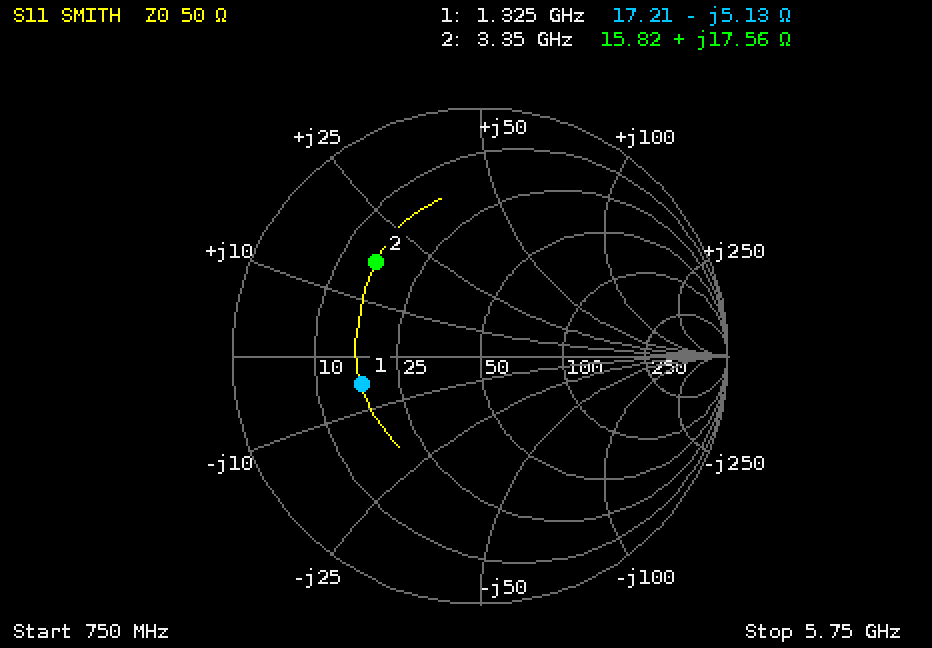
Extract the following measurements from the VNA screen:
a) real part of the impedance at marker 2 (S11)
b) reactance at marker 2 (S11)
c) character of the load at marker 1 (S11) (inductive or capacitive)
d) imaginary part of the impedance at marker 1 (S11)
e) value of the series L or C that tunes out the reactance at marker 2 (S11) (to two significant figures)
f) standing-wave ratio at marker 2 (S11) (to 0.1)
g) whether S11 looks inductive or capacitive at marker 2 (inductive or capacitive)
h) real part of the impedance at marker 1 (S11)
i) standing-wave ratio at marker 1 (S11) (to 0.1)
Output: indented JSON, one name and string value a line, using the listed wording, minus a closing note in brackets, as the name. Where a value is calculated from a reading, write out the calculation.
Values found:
{
  "real part of the impedance at marker 2": "15.82 Ω",
  "reactance at marker 2": "+17.56 Ω",
  "character of the load at marker 1 (S11)": "capacitive",
  "imaginary part of the impedance at marker 1": "-5.13 Ω",
  "value of the series L or C that tunes out the reactance at marker 2 (S11)": "C = 1/(2π × 3.35 GHz × 17.56 Ω) ≈ 2.7 pF",
  "standing-wave ratio at marker 2 (S11)": "3.6",
  "whether S11 looks inductive or capacitive at marker 2": "inductive",
  "real part of the impedance at marker 1": "17.21 Ω",
  "standing-wave ratio at marker 1 (S11)": "2.9"
}
